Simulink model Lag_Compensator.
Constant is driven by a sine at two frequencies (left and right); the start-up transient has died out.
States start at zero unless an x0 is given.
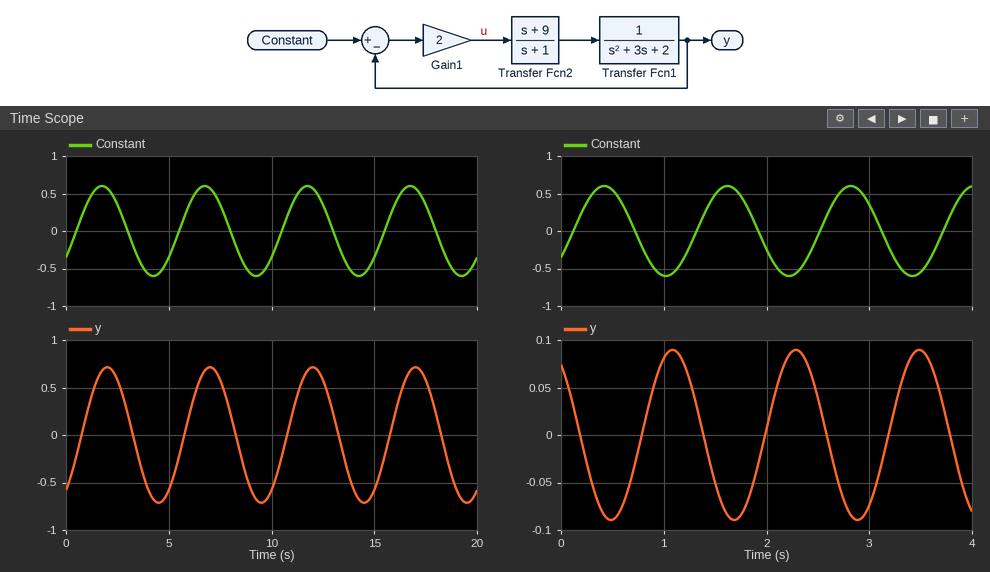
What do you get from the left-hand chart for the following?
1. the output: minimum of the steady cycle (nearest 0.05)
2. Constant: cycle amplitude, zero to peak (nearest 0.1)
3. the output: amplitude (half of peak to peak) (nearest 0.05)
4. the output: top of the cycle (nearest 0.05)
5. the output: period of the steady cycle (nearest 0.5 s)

-0.70
0.6
0.70
0.70
5.0 s
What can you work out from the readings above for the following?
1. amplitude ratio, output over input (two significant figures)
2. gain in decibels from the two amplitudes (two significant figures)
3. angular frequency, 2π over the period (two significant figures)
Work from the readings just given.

1.2
1.3 dB
1.3 rad/s
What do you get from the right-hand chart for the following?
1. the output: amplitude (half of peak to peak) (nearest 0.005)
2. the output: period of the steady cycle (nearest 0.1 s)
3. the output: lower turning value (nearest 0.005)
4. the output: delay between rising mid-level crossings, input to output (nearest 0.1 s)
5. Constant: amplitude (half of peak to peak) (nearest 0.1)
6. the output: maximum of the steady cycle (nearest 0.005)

0.090
1.2 s
-0.090
0.7 s
0.6
0.090
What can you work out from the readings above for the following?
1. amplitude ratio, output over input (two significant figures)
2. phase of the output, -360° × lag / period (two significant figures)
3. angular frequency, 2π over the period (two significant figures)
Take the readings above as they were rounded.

0.15
-210°
5.2 rad/s
